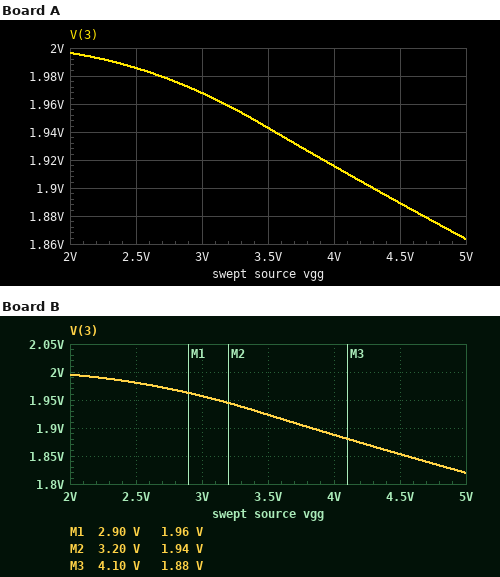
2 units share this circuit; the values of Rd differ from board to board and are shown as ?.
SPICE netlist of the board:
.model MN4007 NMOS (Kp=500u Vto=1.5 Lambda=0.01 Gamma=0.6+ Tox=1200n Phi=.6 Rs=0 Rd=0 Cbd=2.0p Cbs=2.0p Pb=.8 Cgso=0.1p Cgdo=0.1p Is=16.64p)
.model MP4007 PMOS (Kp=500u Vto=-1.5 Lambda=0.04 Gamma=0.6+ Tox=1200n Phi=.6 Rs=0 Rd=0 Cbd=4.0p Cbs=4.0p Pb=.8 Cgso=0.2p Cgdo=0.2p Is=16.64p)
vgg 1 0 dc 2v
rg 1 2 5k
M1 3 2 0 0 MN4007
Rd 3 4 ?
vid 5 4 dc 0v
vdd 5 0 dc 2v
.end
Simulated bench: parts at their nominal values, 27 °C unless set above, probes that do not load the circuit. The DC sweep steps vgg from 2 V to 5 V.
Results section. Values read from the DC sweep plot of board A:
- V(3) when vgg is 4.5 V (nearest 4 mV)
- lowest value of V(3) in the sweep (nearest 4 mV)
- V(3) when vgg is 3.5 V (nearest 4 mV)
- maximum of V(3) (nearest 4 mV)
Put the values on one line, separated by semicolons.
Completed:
1.888 V; 1.864 V; 1.944 V; 1.996 V
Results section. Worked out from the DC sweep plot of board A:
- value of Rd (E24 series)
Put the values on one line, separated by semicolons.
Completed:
56 Ω
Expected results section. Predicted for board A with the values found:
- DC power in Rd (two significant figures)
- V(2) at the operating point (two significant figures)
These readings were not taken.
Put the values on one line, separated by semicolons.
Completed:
230 nW; 2.0 V
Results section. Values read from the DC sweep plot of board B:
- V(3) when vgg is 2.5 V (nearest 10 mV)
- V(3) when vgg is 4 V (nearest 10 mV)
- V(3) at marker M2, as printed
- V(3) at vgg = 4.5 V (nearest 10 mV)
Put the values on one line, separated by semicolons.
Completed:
1.98 V; 1.89 V; 1.94 V; 1.85 V
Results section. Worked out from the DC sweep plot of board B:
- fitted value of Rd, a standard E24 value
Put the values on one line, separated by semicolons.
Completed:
75 Ω
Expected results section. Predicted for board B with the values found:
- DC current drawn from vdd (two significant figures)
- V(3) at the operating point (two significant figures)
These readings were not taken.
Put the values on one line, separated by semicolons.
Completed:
64 µA; 2.0 V
